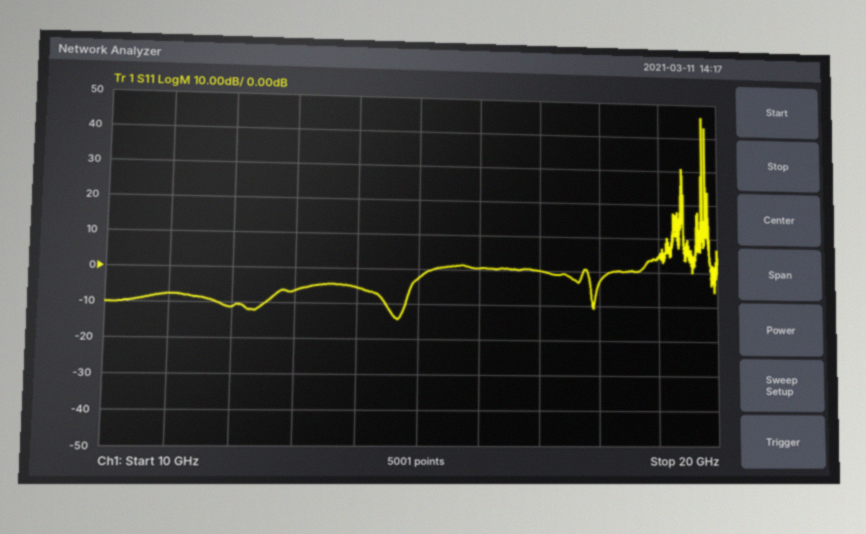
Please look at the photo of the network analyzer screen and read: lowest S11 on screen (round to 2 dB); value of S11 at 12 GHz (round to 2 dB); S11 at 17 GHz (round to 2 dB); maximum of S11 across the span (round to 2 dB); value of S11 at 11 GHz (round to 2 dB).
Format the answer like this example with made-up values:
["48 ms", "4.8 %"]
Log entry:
["-14 dB", "-12 dB", "0 dB", "46 dB", "-8 dB"]
